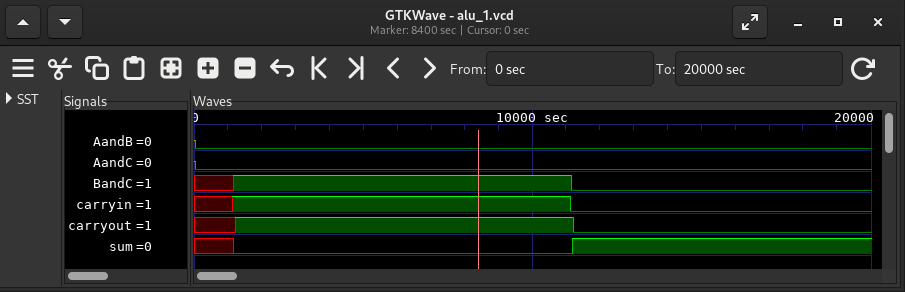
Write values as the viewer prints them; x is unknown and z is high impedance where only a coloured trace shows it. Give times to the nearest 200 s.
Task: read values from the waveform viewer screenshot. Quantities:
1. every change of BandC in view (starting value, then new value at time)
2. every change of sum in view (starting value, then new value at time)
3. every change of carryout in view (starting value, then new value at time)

x, 1 at 1200 s, 0 at 11200 s
x, 0 at 1200 s, 1 at 11200 s
x, 1 at 1200 s, 0 at 11200 s
